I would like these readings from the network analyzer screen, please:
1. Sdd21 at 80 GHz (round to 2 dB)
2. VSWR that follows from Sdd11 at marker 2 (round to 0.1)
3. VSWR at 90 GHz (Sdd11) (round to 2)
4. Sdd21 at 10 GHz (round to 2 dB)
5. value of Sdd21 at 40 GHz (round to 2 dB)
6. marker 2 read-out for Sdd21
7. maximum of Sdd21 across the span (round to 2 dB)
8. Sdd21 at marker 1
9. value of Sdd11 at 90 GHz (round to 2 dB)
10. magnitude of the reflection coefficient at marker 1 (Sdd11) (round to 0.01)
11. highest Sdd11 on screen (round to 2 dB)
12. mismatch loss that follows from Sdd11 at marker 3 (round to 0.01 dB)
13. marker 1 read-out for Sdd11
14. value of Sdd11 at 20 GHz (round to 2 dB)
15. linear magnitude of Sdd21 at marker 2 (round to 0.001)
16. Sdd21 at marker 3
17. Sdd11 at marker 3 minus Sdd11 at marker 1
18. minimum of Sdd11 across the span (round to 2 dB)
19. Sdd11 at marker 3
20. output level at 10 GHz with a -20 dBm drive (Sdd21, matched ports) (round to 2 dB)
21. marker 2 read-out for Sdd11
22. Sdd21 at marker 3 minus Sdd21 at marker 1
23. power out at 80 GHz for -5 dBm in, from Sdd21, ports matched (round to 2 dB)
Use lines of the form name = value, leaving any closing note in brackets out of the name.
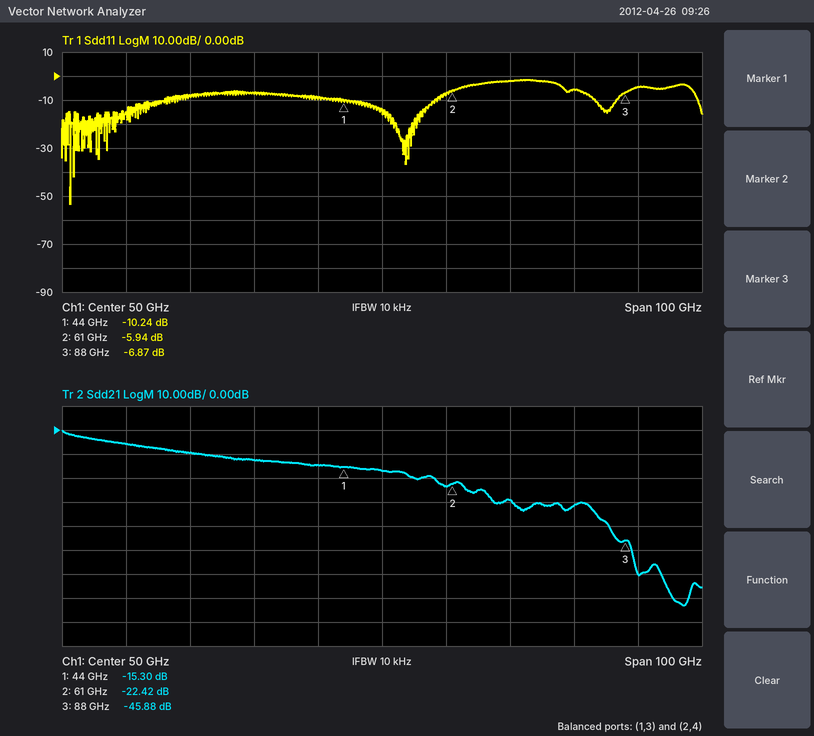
Sdd21 at 80 GHz = -32 dB
VSWR that follows from Sdd11 at marker 2 = 3.0
VSWR at 90 GHz (Sdd11) = 4
Sdd21 at 10 GHz = -6 dB
value of Sdd21 at 40 GHz = -14 dB
marker 2 read-out for Sdd21 = -22.42 dB
maximum of Sdd21 across the span = 0 dB
Sdd21 at marker 1 = -15.30 dB
value of Sdd11 at 90 GHz = -4 dB
magnitude of the reflection coefficient at marker 1 (Sdd11) = 0.31
highest Sdd11 on screen = -2 dB
mismatch loss that follows from Sdd11 at marker 3 = 1.00 dB
marker 1 read-out for Sdd11 = -10.24 dB
value of Sdd11 at 20 GHz = -8 dB
linear magnitude of Sdd21 at marker 2 = 0.076
Sdd21 at marker 3 = -45.88 dB
Sdd11 at marker 3 minus Sdd11 at marker 1 = 3.37 dB
minimum of Sdd11 across the span = -54 dB
Sdd11 at marker 3 = -6.87 dB
output level at 10 GHz with a -20 dBm drive (Sdd21, matched ports) = -26 dBm
marker 2 read-out for Sdd11 = -5.94 dB
Sdd21 at marker 3 minus Sdd21 at marker 1 = -30.58 dB
power out at 80 GHz for -5 dBm in, from Sdd21, ports matched = -36 dBm
